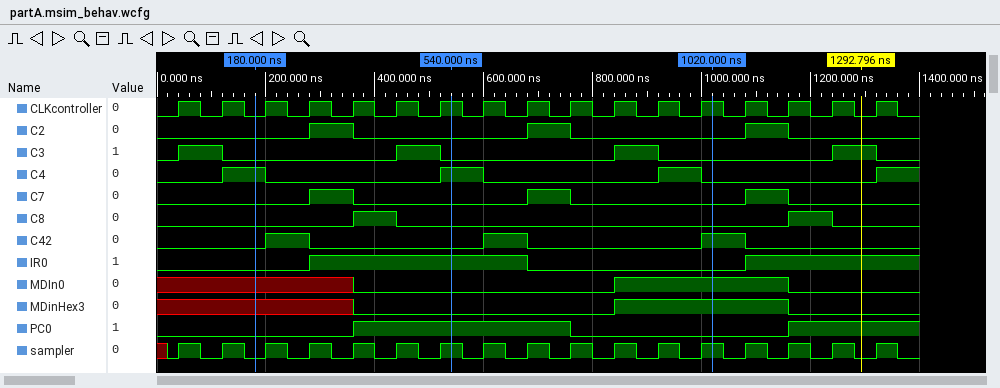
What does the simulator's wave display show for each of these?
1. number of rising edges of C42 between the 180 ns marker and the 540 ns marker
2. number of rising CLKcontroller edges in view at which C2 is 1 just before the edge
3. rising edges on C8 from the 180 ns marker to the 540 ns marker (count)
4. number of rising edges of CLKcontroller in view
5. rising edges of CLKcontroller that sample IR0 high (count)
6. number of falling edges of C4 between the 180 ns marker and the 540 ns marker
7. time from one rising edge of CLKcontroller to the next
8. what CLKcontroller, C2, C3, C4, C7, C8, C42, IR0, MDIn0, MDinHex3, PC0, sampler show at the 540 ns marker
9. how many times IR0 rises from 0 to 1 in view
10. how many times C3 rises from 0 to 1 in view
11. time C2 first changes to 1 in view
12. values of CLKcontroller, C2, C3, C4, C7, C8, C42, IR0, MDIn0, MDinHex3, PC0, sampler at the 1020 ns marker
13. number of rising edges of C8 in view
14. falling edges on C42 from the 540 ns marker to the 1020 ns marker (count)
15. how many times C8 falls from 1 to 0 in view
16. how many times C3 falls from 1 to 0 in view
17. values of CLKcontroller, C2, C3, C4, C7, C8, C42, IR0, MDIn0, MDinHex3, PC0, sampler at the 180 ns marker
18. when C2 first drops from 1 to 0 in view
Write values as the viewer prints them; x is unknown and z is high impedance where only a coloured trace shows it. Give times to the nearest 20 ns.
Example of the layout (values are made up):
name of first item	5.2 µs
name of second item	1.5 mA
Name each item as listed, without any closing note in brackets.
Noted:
number of rising edges of C42 between the 180 ns marker and the 540 ns marker	1
number of rising CLKcontroller edges in view at which C2 is 1 just before the edge	3
rising edges on C8 from the 180 ns marker to the 540 ns marker	1
number of rising edges of CLKcontroller in view	17
rising edges of CLKcontroller that sample IR0 high	8
number of falling edges of C4 between the 180 ns marker and the 540 ns marker	1
time from one rising edge of CLKcontroller to the next	80 ns
what CLKcontroller, C2, C3, C4, C7, C8, C42, IR0, MDIn0, MDinHex3, PC0, sampler show at the 540 ns marker	CLKcontroller=1, C2=0, C3=0, C4=1, C7=0, C8=0, C42=0, IR0=1, MDIn0=0, MDinHex3=0, PC0=1, sampler=1
how many times IR0 rises from 0 to 1 in view	2
how many times C3 rises from 0 to 1 in view	4
time C2 first changes to 1 in view	280 ns
values of CLKcontroller, C2, C3, C4, C7, C8, C42, IR0, MDIn0, MDinHex3, PC0, sampler at the 1020 ns marker	CLKcontroller=1, C2=0, C3=0, C4=0, C7=0, C8=0, C42=1, IR0=0, MDIn0=1, MDinHex3=1, PC0=0, sampler=1
number of rising edges of C8 in view	2
falling edges on C42 from the 540 ns marker to the 1020 ns marker	1
how many times C8 falls from 1 to 0 in view	2
how many times C3 falls from 1 to 0 in view	4
values of CLKcontroller, C2, C3, C4, C7, C8, C42, IR0, MDIn0, MDinHex3, PC0, sampler at the 180 ns marker	CLKcontroller=0, C2=0, C3=0, C4=1, C7=0, C8=0, C42=0, IR0=0, MDIn0=x, MDinHex3=x, PC0=0, sampler=0
when C2 first drops from 1 to 0 in view	360 ns
